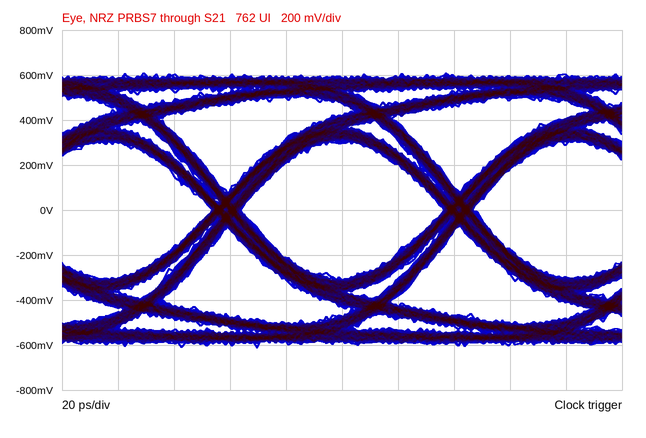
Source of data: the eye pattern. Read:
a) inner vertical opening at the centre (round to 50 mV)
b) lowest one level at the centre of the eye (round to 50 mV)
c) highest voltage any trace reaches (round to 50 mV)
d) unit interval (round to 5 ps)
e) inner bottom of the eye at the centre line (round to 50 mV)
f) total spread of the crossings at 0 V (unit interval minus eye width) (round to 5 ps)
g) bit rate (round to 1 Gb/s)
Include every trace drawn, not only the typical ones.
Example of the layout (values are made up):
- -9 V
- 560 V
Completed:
- 600 mV
- 300 mV
- 600 mV
- 85 ps
- -300 mV
- 10 ps
- 12 Gb/s
